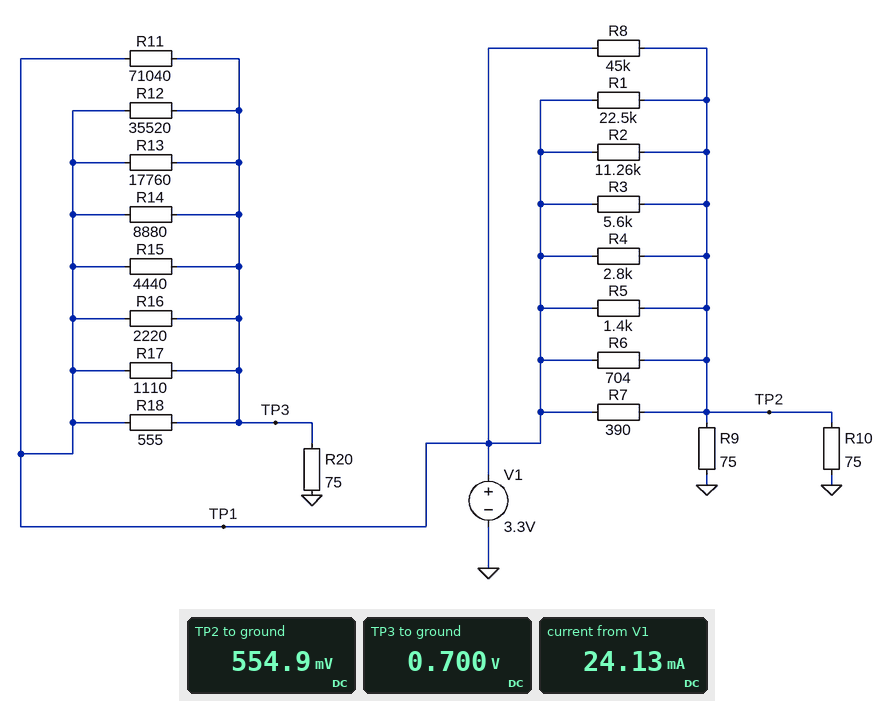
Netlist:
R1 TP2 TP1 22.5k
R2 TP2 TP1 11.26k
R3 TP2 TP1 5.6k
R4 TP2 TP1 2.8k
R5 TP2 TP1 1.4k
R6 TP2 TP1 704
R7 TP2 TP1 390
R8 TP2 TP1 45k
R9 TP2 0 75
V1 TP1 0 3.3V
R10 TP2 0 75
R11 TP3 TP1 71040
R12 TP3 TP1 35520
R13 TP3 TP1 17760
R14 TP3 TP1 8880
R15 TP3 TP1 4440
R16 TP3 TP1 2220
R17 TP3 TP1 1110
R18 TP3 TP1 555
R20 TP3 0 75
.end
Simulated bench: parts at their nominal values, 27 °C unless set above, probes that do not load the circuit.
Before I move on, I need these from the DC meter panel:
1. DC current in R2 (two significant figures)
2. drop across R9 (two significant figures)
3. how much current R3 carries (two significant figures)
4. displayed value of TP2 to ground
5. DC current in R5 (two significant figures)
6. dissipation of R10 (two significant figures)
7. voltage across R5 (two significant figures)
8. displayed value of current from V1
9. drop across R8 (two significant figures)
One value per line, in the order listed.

240 µA
550 mV
490 µA
554.9 mV
2.0 mA
4.1 mW
2.7 V
24.13 mA
2.7 V
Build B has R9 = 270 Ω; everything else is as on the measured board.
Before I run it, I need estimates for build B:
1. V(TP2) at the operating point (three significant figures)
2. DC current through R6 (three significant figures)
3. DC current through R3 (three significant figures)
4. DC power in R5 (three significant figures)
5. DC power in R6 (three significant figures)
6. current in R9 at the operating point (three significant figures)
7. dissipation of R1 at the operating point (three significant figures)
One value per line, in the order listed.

793 mV
3.56 mA
448 µA
4.49 mW
8.93 mW
2.94 mA
279 µW
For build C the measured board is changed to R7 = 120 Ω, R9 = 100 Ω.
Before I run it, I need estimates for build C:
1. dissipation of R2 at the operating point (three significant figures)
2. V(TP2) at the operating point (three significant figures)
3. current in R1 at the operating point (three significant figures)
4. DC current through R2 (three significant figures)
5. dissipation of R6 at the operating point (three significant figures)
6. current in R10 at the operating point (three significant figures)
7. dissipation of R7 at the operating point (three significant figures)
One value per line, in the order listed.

443 µW
1.07 V
99.2 µA
198 µA
7.08 mW
14.2 mA
41.5 mW
